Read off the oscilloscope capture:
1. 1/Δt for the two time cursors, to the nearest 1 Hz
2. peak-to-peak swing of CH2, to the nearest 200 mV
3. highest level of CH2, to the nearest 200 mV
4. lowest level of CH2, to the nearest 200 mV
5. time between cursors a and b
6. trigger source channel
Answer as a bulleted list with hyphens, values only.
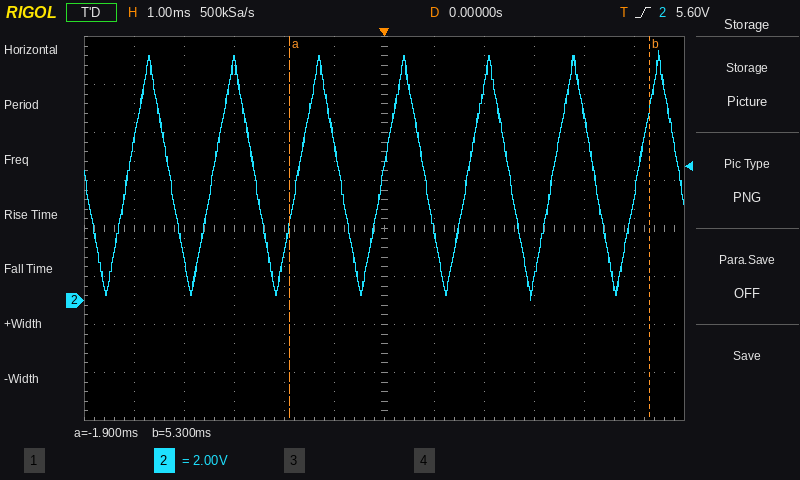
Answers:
- 139 Hz
- 10.4 V
- 10.4 V
- 0.0 V
- 7.2 ms
- CH2
